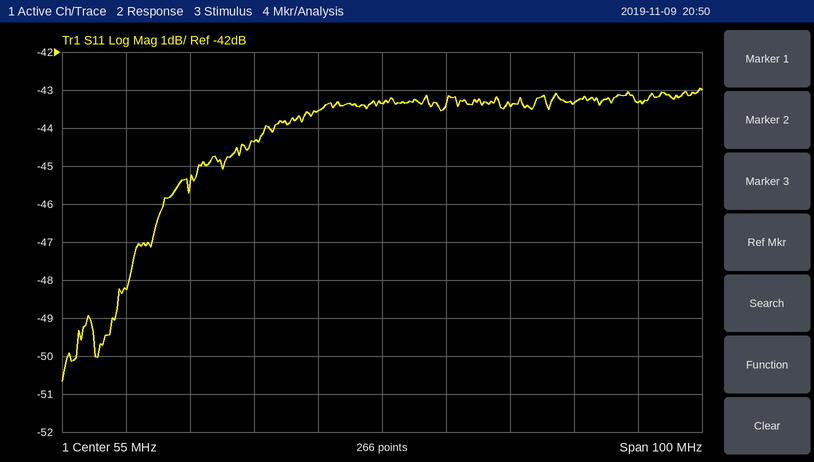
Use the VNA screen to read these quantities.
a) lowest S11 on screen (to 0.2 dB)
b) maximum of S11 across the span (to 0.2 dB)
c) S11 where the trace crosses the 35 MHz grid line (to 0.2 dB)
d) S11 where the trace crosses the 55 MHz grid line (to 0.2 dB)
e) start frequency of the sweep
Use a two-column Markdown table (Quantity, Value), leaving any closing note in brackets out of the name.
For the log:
| Quantity | Value |
|---|---|
| lowest S11 on screen | -50.6 dB |
| maximum of S11 across the span | -43.0 dB |
| S11 where the trace crosses the 35 MHz grid line | -44.4 dB |
| S11 where the trace crosses the 55 MHz grid line | -43.4 dB |
| start frequency of the sweep | 5 MHz |
